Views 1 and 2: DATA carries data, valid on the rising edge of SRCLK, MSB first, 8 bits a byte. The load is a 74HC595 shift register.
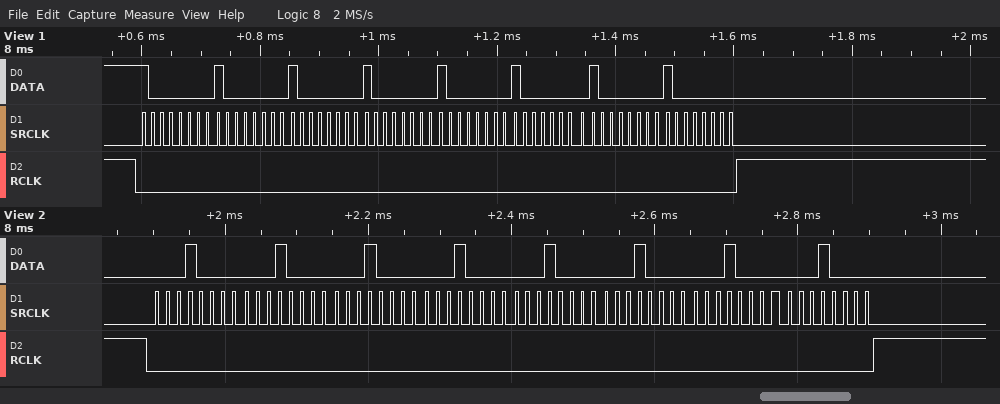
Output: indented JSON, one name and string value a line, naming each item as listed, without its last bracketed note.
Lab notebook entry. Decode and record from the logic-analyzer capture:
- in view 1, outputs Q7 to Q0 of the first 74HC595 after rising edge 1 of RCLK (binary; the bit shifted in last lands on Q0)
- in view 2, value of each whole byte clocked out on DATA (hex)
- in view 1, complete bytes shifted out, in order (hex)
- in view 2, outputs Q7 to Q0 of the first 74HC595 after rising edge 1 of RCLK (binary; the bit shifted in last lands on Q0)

{
  "in view 1, outputs Q7 to Q0 of the first 74HC595 after rising edge 1 of RCLK": "10000000",
  "in view 2, value of each whole byte clocked out on DATA": "0x10 0x10 0x10 0x10 0x10 0x10 0x10 0x10",
  "in view 1, complete bytes shifted out, in order": "80 80 80 80 80 80 80 80",
  "in view 2, outputs Q7 to Q0 of the first 74HC595 after rising edge 1 of RCLK": "00010000"
}
